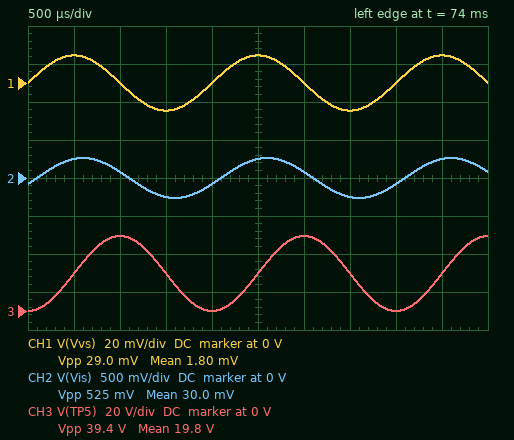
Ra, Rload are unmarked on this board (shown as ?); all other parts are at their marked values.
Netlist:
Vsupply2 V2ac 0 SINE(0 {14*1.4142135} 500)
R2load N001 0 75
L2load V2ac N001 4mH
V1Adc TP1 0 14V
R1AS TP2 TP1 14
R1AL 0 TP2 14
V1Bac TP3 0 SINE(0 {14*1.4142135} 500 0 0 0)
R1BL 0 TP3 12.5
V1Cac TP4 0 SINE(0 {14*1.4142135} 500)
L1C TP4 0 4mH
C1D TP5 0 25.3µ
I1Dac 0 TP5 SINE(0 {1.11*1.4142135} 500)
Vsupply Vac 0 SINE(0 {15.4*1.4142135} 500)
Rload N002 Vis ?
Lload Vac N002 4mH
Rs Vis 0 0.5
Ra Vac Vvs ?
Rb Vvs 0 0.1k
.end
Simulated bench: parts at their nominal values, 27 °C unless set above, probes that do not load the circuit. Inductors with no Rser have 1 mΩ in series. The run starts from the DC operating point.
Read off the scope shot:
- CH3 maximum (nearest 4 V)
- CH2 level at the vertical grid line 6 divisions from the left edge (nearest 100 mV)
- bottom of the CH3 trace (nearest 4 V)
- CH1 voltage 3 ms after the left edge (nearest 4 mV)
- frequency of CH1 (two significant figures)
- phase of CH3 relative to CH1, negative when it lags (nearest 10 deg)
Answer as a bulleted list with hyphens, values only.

- 40 V
- 100 mV
- 0 V
- 0 V
- 500 Hz
- -90 deg
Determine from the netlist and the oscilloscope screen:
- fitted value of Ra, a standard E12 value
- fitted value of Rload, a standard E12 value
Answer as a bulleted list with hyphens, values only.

- 150 kΩ
- 39 Ω
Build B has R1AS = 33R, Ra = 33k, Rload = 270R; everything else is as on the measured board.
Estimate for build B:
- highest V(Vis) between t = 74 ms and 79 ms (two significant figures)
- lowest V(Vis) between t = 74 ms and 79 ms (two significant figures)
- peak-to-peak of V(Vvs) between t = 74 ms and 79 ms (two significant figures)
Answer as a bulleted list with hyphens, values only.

- 40 mV
- -40 mV
- 130 mV
